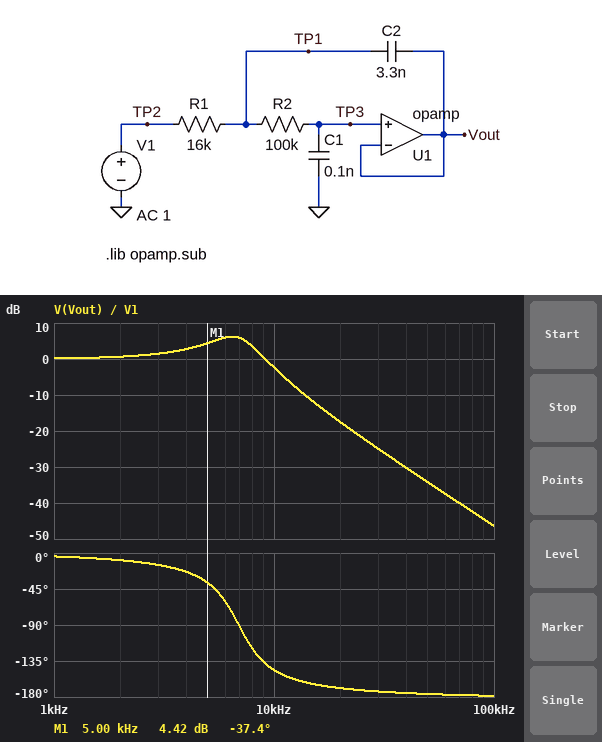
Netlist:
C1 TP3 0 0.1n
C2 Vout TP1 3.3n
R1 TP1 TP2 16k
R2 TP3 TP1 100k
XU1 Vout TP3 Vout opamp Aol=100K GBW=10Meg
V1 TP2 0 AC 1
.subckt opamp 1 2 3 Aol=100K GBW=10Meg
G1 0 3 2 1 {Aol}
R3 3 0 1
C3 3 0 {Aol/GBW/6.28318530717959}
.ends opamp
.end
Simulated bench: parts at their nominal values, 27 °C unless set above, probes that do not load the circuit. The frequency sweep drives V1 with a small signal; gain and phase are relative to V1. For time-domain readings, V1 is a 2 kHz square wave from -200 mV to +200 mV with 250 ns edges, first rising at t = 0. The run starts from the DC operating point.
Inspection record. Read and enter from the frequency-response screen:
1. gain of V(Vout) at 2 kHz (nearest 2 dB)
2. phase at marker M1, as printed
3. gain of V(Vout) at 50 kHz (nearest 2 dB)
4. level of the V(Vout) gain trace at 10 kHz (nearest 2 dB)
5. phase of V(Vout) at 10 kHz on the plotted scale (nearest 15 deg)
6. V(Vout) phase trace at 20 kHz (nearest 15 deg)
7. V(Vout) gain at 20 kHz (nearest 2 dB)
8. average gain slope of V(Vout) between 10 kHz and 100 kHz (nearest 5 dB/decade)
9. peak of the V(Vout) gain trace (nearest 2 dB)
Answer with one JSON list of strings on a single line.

["0 dB", "-37.4 deg", "-34 dB", "-2 dB", "-150 deg", "-165 deg", "-18 dB", "-45 dB/decade", "6 dB"]
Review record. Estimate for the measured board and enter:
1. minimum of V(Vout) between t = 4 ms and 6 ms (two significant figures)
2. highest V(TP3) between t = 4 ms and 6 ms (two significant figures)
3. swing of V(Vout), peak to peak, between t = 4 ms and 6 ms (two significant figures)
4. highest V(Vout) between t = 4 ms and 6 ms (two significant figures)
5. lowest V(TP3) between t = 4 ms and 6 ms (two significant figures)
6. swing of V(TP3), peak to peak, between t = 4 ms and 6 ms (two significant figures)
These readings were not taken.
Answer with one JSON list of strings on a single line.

["-380 mV", "380 mV", "770 mV", "380 mV", "-380 mV", "770 mV"]
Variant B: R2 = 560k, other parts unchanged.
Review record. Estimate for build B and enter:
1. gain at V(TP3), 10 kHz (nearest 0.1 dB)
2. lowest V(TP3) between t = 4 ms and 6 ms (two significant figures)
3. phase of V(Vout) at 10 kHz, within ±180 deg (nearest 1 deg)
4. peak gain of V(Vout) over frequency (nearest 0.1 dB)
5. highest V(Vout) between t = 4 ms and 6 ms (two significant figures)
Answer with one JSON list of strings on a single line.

["-21.0 dB", "-260 mV", "-161 deg", "0.9 dB", "260 mV"]
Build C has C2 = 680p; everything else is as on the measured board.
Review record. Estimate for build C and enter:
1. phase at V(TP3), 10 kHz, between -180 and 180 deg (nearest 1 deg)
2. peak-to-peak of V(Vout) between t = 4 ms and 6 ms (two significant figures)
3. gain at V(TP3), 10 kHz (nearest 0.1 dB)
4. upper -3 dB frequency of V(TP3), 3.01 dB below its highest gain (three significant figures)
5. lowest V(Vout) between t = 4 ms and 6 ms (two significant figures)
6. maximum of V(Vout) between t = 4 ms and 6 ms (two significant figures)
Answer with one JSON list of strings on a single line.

["-52 deg", "500 mV", "0.7 dB", "17.4 kHz", "-250 mV", "250 mV"]
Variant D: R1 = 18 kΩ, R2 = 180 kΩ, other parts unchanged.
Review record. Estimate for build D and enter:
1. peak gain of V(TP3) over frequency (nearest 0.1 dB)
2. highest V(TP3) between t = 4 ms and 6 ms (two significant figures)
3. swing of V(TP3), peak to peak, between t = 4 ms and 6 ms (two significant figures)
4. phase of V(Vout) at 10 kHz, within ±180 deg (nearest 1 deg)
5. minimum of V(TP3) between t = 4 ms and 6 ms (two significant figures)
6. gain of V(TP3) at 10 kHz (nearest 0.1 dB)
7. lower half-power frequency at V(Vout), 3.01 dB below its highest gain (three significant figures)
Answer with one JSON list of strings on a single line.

["4.8 dB", "340 mV", "670 mV", "-159 deg", "-340 mV", "-10.8 dB", "2.38 kHz"]
